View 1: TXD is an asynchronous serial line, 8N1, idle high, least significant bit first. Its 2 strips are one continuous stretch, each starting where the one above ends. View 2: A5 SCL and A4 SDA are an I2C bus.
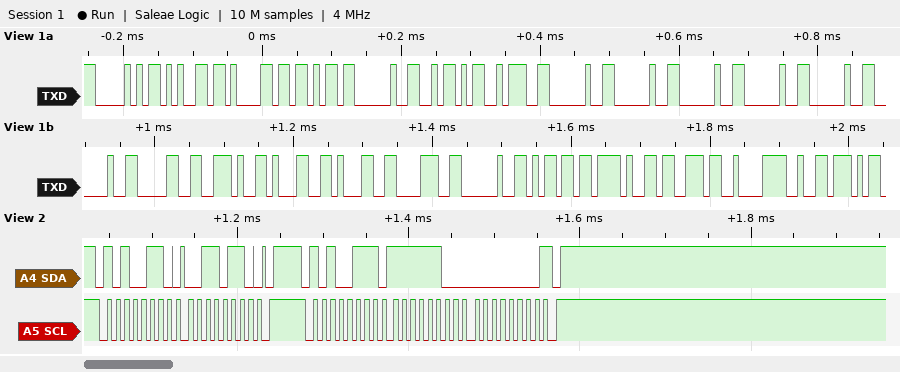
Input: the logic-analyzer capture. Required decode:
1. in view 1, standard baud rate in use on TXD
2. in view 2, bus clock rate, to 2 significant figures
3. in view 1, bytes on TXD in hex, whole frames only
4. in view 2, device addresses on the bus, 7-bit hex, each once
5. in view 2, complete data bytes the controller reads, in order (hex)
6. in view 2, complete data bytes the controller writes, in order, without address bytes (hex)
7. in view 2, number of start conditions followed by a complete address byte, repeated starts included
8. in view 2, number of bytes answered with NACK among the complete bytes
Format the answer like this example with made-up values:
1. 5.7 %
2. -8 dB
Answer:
1. 115200 baud
2. 100 kHz
3. 50 65 61 6B 20 5A 3A 20 20 20 20 20 20 30 2E 31 31 38 20 6D 2F 73 C2 B2
4. 0x53
5. FC 00
6. 36
7. 2
8. 1
